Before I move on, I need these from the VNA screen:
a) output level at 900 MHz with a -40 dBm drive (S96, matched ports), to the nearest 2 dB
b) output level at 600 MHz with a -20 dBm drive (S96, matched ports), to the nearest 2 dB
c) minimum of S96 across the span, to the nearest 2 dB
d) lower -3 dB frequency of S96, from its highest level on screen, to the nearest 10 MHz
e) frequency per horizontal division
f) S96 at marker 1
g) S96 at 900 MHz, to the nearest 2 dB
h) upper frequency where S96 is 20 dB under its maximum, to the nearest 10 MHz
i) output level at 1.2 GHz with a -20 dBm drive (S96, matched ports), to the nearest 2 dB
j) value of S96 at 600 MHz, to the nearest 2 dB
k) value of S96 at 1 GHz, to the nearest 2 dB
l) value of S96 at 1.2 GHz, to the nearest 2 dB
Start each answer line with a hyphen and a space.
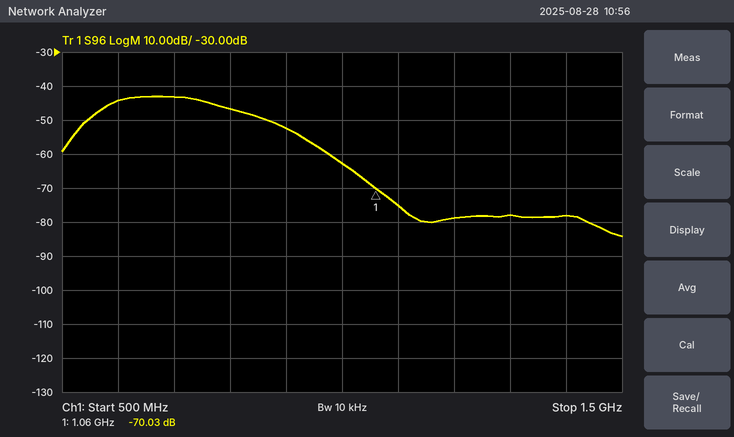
- -92 dBm
- -64 dBm
- -84 dB
- 580 MHz
- 100 MHz
- -70.03 dB
- -52 dB
- 1.00 GHz
- -98 dBm
- -44 dB
- -62 dB
- -78 dB
